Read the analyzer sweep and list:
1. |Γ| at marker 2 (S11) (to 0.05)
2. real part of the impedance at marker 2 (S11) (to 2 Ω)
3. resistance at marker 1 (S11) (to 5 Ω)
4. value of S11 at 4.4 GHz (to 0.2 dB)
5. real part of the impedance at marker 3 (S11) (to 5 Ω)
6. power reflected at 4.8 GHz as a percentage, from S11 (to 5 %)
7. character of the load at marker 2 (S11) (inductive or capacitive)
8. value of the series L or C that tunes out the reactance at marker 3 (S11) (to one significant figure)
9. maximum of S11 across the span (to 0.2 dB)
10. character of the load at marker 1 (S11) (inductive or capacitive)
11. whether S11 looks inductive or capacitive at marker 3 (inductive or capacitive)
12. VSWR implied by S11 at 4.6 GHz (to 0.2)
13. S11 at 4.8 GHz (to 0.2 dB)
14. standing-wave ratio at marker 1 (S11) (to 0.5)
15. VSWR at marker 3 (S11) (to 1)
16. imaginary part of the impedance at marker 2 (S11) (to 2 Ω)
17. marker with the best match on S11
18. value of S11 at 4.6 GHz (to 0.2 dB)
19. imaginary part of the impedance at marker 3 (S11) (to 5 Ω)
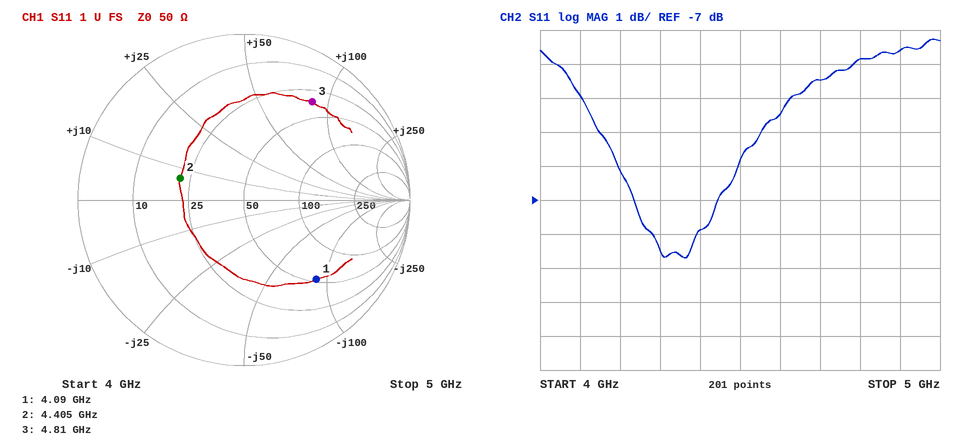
0.40
22 Ω
55 Ω
-7.8 dB
35 Ω
50 %
inductive
400 fF
-2.2 dB
capacitive
inductive
4.0
-2.8 dB
4.5
6
+6 Ω
marker 2
-4.4 dB
+85 Ω
